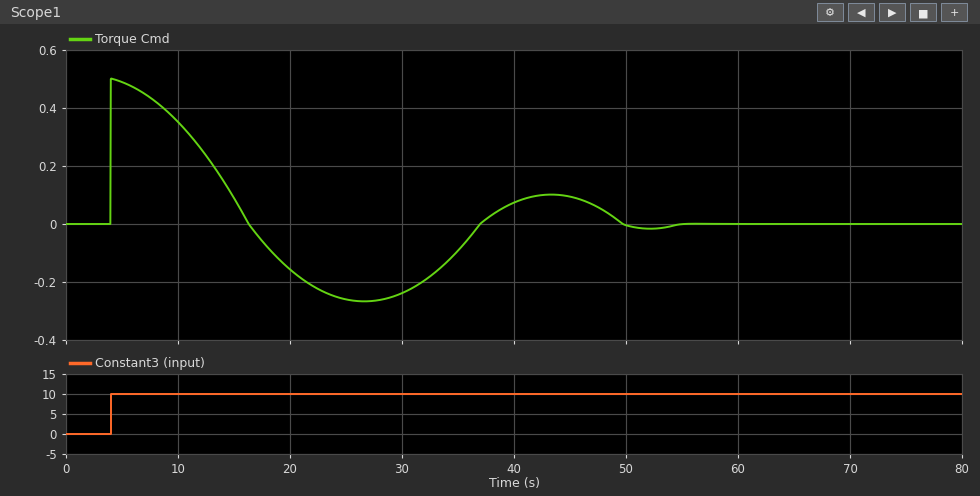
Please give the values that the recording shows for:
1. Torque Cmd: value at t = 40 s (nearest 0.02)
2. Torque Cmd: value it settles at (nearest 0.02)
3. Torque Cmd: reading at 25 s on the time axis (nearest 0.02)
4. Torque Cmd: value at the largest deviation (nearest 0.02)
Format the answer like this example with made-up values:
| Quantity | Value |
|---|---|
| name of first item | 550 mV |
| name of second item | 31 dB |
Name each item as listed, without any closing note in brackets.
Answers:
| Quantity | Value |
|---|---|
| Torque Cmd: value at t = 40 s | 0.08 |
| Torque Cmd: value it settles at | 0.00 |
| Torque Cmd: reading at 25 s on the time axis | -0.26 |
| Torque Cmd: value at the largest deviation | 0.50 |
